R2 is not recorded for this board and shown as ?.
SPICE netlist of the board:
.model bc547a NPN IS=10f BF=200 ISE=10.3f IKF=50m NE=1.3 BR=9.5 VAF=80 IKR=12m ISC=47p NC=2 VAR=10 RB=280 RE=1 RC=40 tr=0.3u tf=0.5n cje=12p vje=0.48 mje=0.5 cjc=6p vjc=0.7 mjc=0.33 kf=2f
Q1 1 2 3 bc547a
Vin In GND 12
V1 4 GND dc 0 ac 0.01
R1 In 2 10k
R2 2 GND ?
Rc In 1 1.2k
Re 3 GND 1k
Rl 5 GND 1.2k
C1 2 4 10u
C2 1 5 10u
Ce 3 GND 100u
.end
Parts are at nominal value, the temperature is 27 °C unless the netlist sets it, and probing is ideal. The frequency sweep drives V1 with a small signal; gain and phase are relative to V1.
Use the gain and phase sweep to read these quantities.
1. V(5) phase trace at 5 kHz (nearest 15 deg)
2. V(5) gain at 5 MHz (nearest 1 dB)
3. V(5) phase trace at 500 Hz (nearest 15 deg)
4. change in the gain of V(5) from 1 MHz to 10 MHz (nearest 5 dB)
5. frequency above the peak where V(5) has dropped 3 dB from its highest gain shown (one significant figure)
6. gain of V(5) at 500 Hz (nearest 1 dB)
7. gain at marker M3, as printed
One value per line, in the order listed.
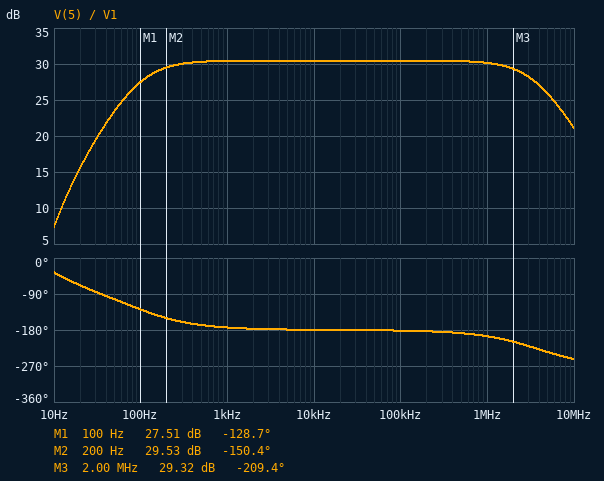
-180 deg
26 dB
-165 deg
-10 dB
4 MHz
30 dB
29.32 dB
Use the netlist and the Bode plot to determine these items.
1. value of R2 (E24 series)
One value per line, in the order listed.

2.7 kΩ
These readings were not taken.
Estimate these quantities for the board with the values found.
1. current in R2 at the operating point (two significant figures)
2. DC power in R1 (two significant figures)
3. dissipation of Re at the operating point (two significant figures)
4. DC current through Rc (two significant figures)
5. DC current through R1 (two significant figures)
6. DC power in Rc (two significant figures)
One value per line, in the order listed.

930 µA
9.0 mW
3.4 mW
1.8 mA
950 µA
4.0 mW
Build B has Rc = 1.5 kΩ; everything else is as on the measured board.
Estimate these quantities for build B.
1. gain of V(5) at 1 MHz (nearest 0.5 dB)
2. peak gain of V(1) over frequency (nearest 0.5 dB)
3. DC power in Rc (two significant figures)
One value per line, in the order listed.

31.0 dB
31.5 dB
5.0 mW
